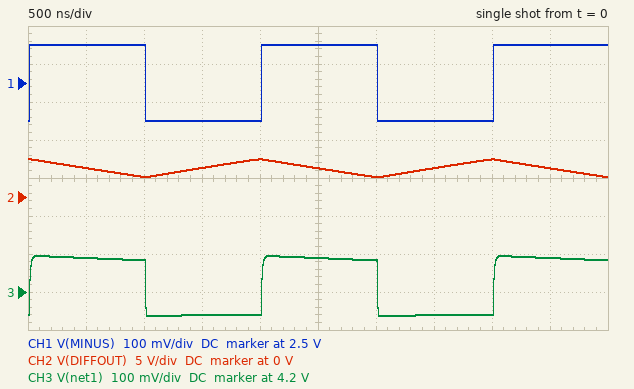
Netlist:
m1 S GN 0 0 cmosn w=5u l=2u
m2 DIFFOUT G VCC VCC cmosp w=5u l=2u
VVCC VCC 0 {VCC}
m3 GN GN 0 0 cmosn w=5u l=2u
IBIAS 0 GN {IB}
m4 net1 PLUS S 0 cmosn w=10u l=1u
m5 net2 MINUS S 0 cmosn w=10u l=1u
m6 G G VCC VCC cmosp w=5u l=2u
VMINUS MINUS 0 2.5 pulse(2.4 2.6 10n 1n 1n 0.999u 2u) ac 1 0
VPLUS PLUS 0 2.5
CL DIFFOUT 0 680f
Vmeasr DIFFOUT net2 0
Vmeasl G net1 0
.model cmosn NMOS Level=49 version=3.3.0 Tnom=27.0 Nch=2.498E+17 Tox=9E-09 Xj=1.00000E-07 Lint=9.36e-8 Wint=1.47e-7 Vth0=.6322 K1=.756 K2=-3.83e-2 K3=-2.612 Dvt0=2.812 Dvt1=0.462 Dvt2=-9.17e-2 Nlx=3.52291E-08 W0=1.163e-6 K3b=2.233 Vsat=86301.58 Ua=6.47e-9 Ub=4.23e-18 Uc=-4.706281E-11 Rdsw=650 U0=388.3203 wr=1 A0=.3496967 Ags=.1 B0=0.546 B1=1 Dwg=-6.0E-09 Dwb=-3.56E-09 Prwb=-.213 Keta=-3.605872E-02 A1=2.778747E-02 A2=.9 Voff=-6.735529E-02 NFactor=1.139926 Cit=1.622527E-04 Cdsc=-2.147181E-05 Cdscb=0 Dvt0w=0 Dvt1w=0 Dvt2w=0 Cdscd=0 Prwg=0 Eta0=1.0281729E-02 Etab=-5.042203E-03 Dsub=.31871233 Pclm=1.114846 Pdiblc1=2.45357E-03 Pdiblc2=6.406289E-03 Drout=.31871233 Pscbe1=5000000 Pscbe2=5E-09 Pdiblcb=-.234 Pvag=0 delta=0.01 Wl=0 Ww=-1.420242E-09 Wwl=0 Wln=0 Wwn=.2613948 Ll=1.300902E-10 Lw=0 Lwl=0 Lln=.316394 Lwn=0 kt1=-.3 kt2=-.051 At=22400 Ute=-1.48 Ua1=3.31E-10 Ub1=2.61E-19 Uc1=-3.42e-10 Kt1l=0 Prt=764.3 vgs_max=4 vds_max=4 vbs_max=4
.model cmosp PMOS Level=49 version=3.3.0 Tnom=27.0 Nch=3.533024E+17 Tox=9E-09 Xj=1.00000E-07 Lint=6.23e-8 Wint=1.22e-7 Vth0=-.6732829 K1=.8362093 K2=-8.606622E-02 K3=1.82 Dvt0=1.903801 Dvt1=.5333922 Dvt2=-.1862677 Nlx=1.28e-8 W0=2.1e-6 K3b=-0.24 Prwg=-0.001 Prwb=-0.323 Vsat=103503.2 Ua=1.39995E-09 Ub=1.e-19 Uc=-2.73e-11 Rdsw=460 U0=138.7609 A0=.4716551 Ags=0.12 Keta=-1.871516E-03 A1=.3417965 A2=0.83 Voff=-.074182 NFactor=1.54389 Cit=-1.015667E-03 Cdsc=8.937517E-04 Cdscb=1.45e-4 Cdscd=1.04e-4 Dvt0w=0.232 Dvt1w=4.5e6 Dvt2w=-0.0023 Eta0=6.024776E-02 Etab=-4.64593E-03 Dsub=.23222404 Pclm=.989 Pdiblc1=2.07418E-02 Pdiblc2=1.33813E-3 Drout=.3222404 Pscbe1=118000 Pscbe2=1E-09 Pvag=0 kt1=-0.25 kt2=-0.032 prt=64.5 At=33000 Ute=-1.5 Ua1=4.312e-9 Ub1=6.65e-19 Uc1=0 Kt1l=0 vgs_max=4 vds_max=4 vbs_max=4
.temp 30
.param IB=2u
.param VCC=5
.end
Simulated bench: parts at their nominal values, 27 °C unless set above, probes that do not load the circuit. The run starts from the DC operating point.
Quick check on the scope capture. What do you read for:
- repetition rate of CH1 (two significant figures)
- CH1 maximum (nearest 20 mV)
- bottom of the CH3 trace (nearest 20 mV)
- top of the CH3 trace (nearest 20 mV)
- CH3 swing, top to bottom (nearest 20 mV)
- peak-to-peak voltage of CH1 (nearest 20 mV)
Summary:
500 kHz
2.60 V
4.14 V
4.30 V
160 mV
200 mV
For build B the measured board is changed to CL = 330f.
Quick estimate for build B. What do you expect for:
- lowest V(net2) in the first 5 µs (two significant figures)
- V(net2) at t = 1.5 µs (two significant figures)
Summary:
1.5 V
4.0 V
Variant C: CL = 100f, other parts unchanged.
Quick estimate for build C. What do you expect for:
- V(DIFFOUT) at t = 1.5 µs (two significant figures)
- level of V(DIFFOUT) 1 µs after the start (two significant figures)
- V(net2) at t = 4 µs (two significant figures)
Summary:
5.0 V
1.5 V
5.0 V
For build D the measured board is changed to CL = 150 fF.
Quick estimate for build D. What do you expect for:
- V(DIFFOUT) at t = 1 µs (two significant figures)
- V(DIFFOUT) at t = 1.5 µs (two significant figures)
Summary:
1.5 V
5.0 V
